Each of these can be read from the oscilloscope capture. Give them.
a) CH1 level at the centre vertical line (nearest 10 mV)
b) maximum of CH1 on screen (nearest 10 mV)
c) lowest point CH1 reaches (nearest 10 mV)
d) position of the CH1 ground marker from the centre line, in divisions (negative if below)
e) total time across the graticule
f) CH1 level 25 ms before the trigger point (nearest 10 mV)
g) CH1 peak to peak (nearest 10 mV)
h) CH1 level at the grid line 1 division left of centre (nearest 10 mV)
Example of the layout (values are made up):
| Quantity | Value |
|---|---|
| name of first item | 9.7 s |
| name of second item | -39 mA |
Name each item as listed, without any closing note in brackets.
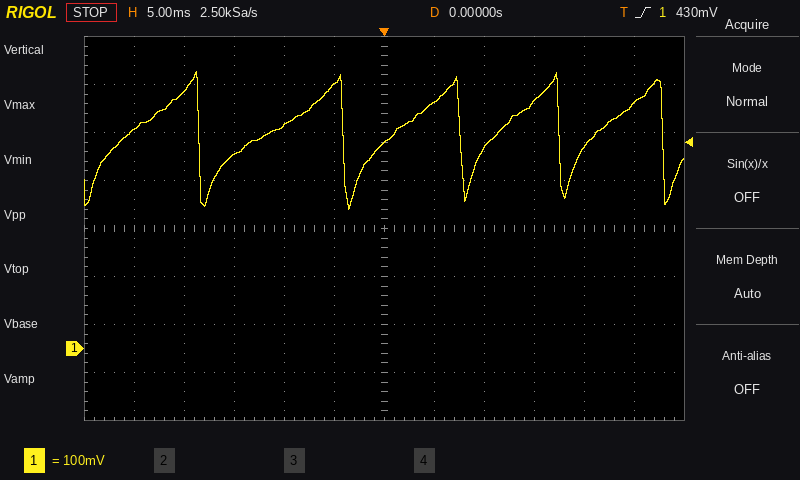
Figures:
| Quantity | Value |
|---|---|
| CH1 level at the centre vertical line | 430 mV |
| maximum of CH1 on screen | 580 mV |
| lowest point CH1 reaches | 290 mV |
| position of the CH1 ground marker from the centre line, in divisions | -2.5 div |
| total time across the graticule | 60 ms |
| CH1 level 25 ms before the trigger point | 460 mV |
| CH1 peak to peak | 290 mV |
| CH1 level at the grid line 1 division left of centre | 550 mV |
